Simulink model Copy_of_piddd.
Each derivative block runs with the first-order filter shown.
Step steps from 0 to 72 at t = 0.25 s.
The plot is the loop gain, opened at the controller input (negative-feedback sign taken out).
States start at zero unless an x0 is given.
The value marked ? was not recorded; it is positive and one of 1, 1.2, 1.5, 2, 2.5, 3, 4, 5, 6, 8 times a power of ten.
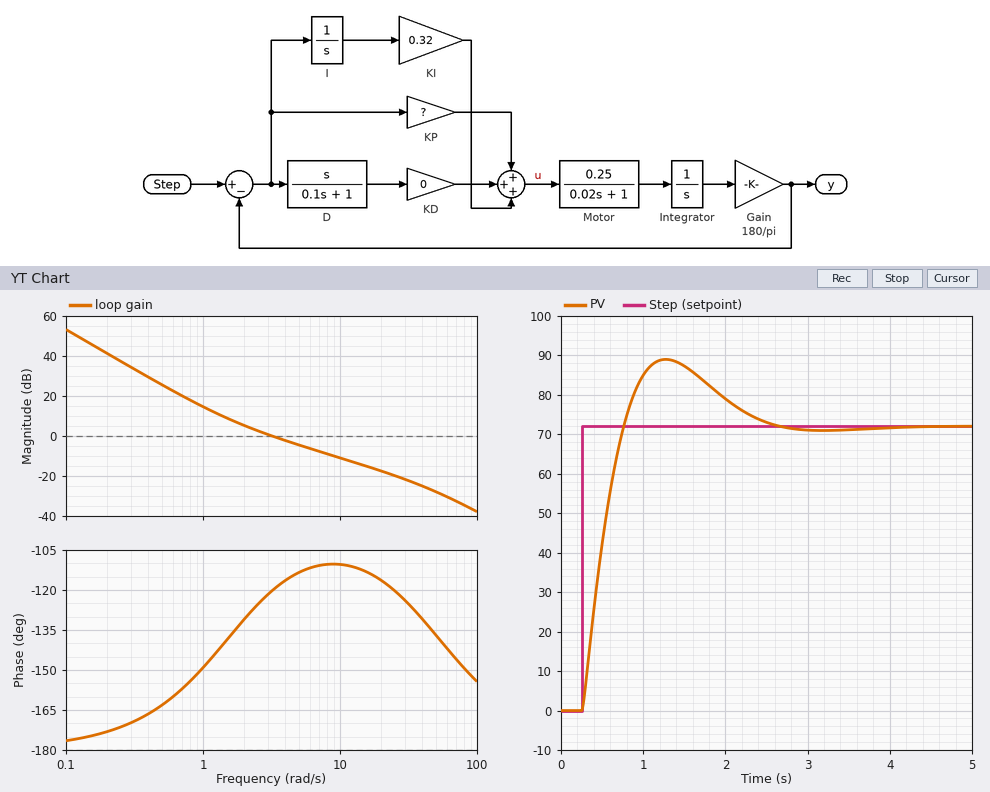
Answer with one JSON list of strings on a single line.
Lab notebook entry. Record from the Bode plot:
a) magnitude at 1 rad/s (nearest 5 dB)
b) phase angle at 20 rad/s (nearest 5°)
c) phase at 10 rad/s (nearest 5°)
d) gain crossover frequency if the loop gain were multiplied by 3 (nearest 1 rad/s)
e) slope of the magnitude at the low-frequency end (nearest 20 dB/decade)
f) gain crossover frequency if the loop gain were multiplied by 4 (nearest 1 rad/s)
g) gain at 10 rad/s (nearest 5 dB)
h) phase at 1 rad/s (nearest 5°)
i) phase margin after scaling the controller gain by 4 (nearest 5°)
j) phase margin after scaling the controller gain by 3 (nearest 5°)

["15 dB", "-115°", "-110°", "9 rad/s", "-40 dB/decade", "11 rad/s", "-10 dB", "-150°", "70°", "70°"]
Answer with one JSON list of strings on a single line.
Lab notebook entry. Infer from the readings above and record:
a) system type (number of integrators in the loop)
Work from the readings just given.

["2"]
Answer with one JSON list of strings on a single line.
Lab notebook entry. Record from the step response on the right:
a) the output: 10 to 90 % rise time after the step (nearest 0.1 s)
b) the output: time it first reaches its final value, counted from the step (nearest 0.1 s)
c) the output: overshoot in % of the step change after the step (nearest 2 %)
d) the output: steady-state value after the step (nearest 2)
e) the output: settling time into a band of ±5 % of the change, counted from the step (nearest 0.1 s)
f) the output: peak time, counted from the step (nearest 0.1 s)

["0.4 s", "0.5 s", "24 %", "72", "2.0 s", "1.0 s"]
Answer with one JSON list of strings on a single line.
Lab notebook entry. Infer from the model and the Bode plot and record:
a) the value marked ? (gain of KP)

["0.2"]
